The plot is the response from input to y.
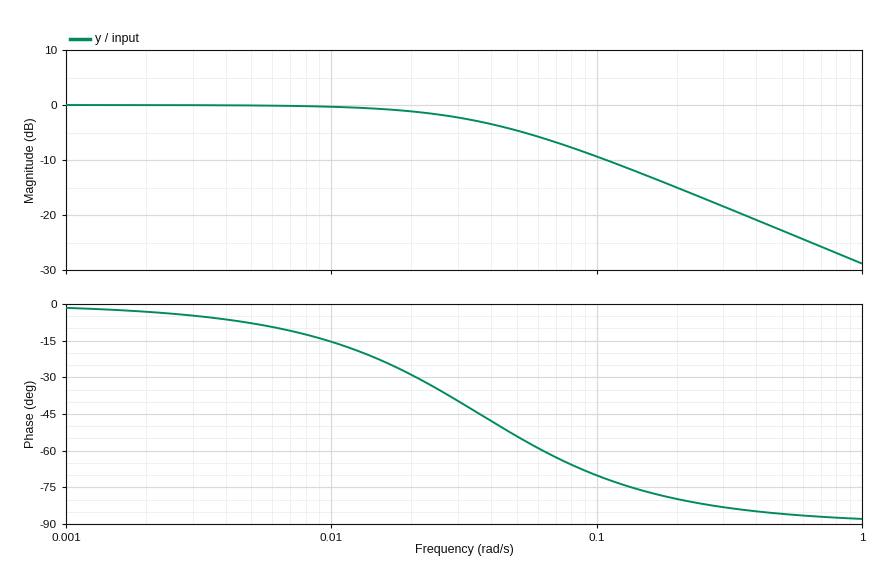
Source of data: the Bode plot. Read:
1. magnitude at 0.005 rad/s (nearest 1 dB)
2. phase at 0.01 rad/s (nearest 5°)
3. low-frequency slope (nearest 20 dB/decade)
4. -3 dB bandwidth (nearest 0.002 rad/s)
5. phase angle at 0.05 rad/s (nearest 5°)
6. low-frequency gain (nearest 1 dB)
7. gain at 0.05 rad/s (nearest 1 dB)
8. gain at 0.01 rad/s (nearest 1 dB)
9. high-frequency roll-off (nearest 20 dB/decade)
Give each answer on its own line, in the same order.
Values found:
0 dB
-15°
0 dB/decade
0.036 rad/s
-55°
0 dB
-5 dB
0 dB
-20 dB/decade
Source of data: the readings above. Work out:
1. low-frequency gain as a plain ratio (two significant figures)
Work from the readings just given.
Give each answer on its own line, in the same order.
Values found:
1.0
